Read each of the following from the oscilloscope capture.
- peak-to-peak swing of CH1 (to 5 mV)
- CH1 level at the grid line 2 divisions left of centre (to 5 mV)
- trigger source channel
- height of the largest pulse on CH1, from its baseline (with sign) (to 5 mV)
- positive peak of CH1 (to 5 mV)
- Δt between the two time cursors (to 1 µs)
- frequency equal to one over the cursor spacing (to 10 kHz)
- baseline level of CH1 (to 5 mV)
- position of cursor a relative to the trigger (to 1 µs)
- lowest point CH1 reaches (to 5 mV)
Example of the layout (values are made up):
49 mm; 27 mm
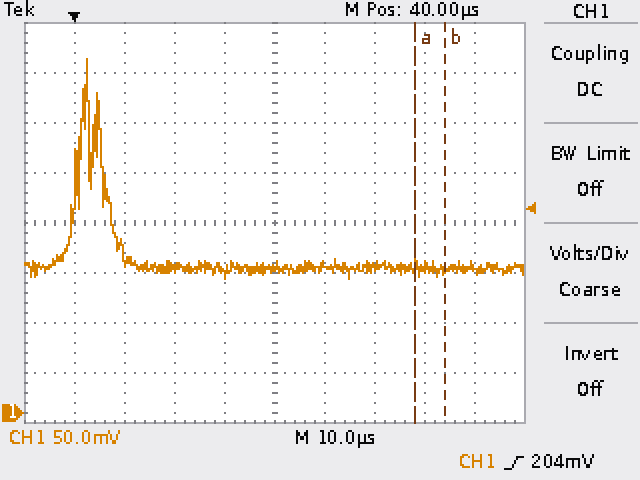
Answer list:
220 mV; 145 mV; CH1; +210 mV; 355 mV; 6 µs; 170 kHz; 145 mV; +68 µs; 135 mV
